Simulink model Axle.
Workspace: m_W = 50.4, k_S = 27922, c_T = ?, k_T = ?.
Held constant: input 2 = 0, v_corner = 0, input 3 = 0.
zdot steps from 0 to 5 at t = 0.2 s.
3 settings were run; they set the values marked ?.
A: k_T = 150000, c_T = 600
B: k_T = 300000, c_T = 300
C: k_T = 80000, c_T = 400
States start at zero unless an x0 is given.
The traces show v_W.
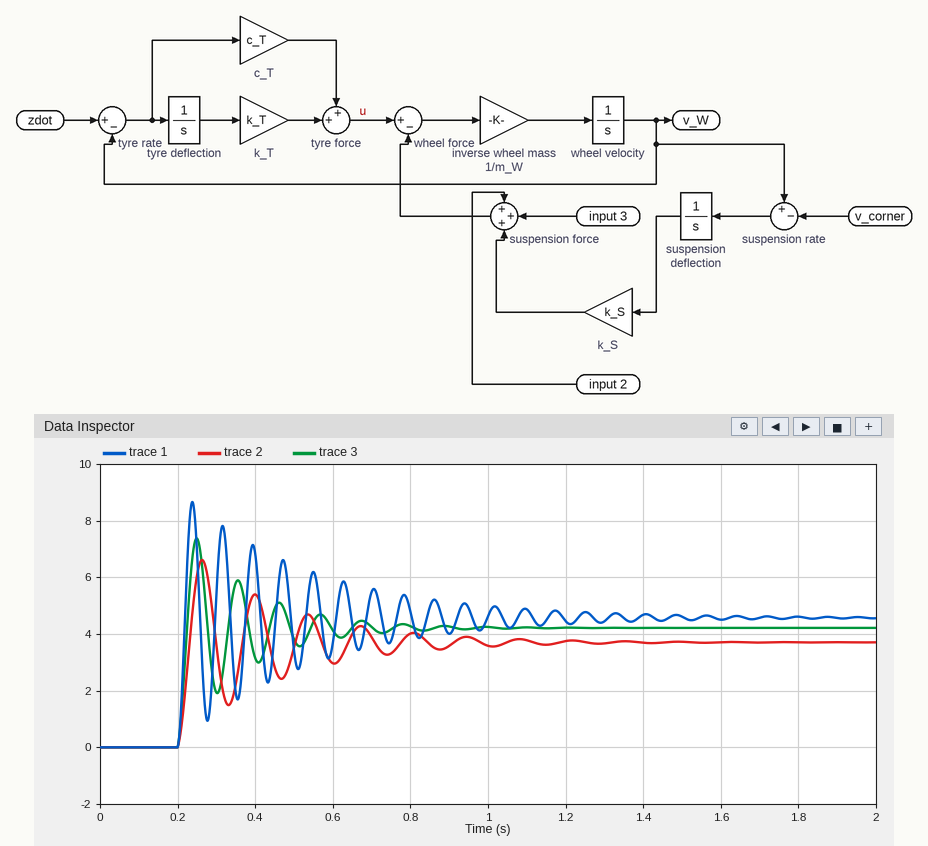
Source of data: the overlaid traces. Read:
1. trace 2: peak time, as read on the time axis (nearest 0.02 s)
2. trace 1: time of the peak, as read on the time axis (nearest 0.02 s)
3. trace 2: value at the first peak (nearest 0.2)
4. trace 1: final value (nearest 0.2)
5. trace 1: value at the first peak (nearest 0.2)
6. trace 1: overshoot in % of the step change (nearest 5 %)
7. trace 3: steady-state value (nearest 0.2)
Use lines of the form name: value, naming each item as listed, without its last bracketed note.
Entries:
trace 2: peak time, as read on the time axis: 0.26 s
trace 1: time of the peak, as read on the time axis: 0.24 s
trace 2: value at the first peak: 6.6
trace 1: final value: 4.6
trace 1: value at the first peak: 8.6
trace 1: overshoot in % of the step change: 90 %
trace 3: steady-state value: 4.2
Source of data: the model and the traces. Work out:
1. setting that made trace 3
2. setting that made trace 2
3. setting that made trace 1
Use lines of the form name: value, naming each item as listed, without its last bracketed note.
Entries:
setting that made trace 3: A
setting that made trace 2: C
setting that made trace 1: B
